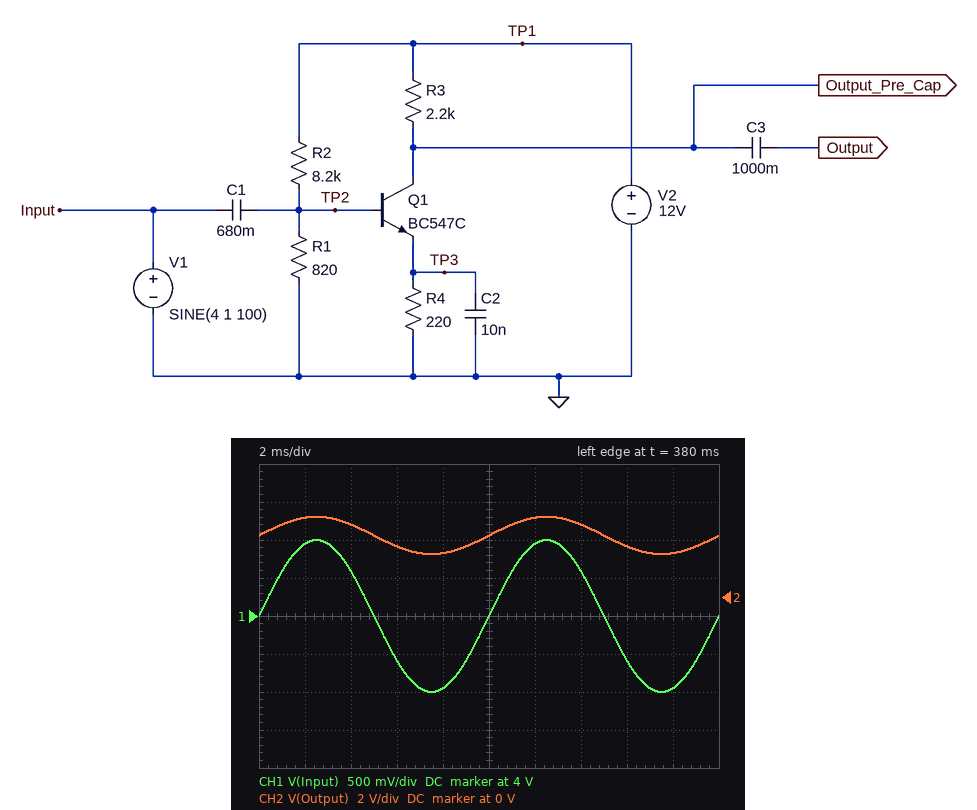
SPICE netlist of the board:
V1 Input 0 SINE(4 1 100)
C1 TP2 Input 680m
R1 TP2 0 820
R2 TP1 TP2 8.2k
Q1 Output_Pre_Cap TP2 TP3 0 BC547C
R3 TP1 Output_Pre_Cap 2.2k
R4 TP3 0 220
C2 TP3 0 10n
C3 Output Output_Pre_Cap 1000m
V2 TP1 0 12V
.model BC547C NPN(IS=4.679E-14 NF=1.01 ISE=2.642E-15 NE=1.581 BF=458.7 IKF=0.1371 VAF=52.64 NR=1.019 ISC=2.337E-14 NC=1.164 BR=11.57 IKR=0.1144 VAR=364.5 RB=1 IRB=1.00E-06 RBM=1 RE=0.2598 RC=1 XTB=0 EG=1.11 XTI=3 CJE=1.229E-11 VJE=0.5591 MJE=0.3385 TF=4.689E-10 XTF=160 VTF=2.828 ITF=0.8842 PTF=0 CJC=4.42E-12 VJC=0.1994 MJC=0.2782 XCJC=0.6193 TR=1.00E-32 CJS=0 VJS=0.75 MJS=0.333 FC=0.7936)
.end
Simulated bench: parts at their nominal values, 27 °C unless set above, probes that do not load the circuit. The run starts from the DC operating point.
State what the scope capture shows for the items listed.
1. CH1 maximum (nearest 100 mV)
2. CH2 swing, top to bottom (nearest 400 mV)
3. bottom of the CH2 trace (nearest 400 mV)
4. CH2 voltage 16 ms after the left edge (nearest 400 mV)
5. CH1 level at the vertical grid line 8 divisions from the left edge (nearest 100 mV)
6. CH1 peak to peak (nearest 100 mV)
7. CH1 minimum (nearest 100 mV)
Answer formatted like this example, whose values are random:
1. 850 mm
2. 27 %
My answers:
1. 5.0 V
2. 2.0 V
3. 2.4 V
4. 2.8 V
5. 3.4 V
6. 2.0 V
7. 3.0 V
